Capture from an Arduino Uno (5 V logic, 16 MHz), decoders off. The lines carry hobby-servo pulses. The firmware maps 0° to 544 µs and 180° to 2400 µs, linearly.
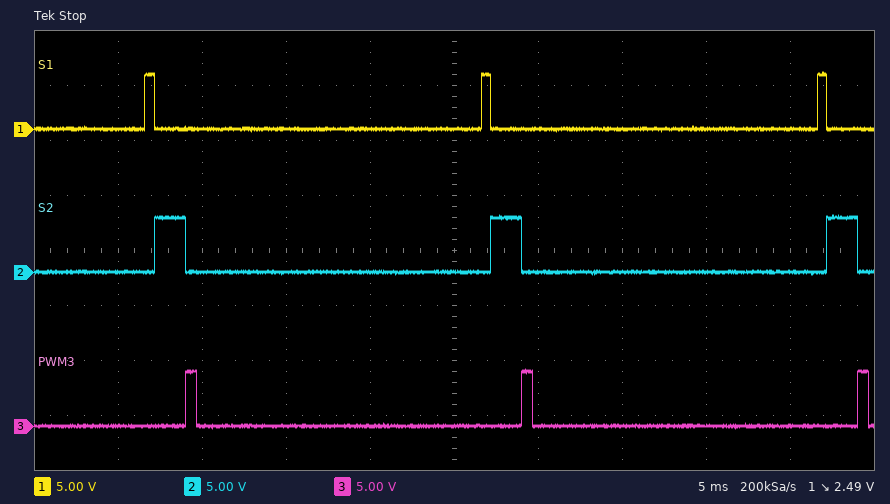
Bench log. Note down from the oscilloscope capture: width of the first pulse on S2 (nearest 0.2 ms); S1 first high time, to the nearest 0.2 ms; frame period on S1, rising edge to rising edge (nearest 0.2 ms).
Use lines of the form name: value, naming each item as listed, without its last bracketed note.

width of the first pulse on S2: 1.8 ms
S1 first high time, to the nearest 0.2 ms: 0.6 ms
frame period on S1, rising edge to rising edge: 20.0 ms
